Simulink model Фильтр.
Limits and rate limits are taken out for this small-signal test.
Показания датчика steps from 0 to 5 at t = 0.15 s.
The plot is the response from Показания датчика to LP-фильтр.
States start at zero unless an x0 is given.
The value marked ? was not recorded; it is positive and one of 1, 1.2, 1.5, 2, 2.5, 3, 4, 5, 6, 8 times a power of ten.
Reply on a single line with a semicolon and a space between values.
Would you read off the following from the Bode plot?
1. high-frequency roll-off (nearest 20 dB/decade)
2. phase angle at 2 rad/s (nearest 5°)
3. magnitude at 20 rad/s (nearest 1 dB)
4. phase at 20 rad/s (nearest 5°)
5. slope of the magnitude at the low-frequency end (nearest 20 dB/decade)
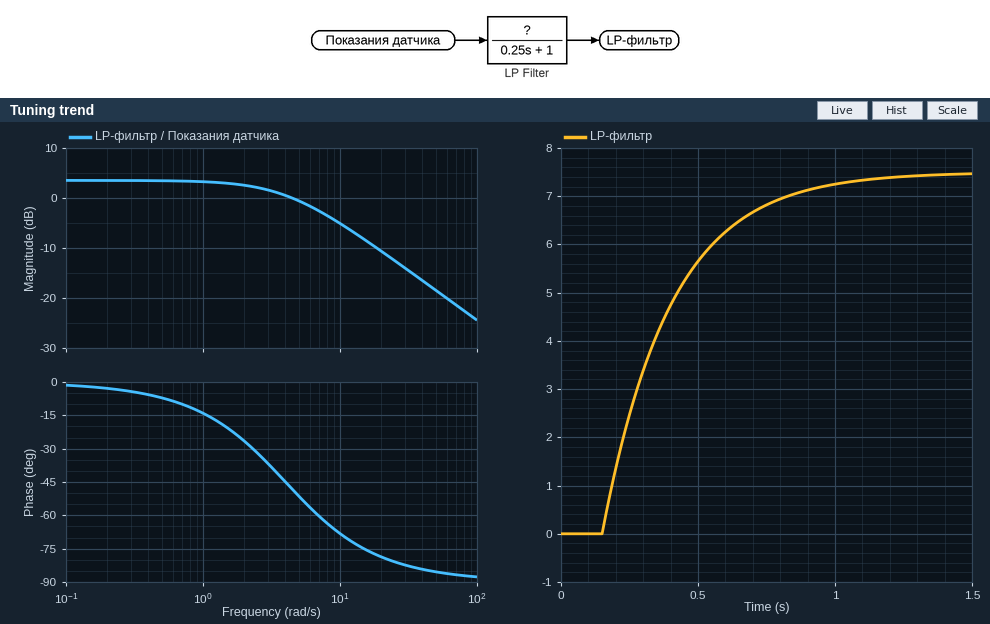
-20 dB/decade; -25°; -11 dB; -80°; 0 dB/decade
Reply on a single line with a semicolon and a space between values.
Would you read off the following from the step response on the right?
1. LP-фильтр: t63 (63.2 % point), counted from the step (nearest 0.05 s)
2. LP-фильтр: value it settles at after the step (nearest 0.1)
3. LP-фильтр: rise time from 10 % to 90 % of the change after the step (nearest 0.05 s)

0.25 s; 7.5; 0.55 s
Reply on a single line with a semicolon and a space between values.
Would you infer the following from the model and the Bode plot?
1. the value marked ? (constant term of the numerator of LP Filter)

1.5
